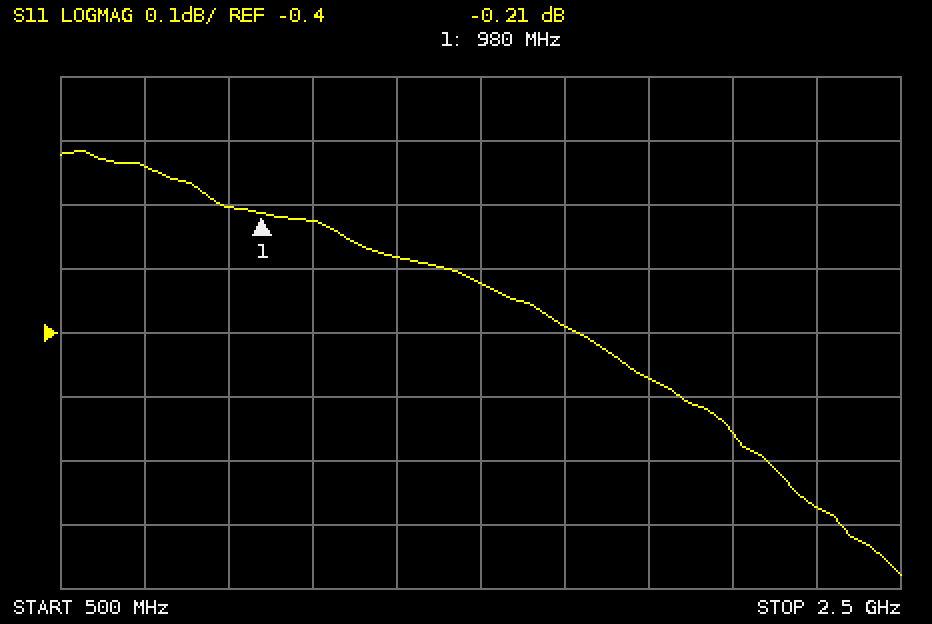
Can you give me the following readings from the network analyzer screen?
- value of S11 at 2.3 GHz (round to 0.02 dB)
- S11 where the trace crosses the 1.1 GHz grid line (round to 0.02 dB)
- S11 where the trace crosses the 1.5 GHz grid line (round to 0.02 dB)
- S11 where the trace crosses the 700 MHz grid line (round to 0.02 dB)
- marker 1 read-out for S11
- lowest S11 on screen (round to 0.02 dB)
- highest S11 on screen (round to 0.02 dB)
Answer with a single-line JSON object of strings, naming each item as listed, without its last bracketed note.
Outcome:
{"value of S11 at 2.3 GHz": "-0.68 dB", "S11 where the trace crosses the 1.1 GHz grid line": "-0.22 dB", "S11 where the trace crosses the 1.5 GHz grid line": "-0.32 dB", "S11 where the trace crosses the 700 MHz grid line": "-0.14 dB", "marker 1 read-out for S11": "-0.21 dB", "lowest S11 on screen": "-0.78 dB", "highest S11 on screen": "-0.12 dB"}
